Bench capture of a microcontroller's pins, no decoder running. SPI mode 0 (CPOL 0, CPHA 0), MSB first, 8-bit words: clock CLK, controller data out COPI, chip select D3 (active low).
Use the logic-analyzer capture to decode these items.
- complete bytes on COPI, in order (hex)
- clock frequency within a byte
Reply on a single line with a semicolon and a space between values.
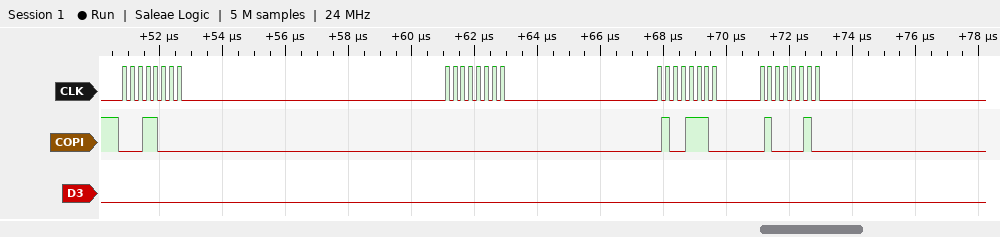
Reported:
18 00 4E 42; 4 MHz
